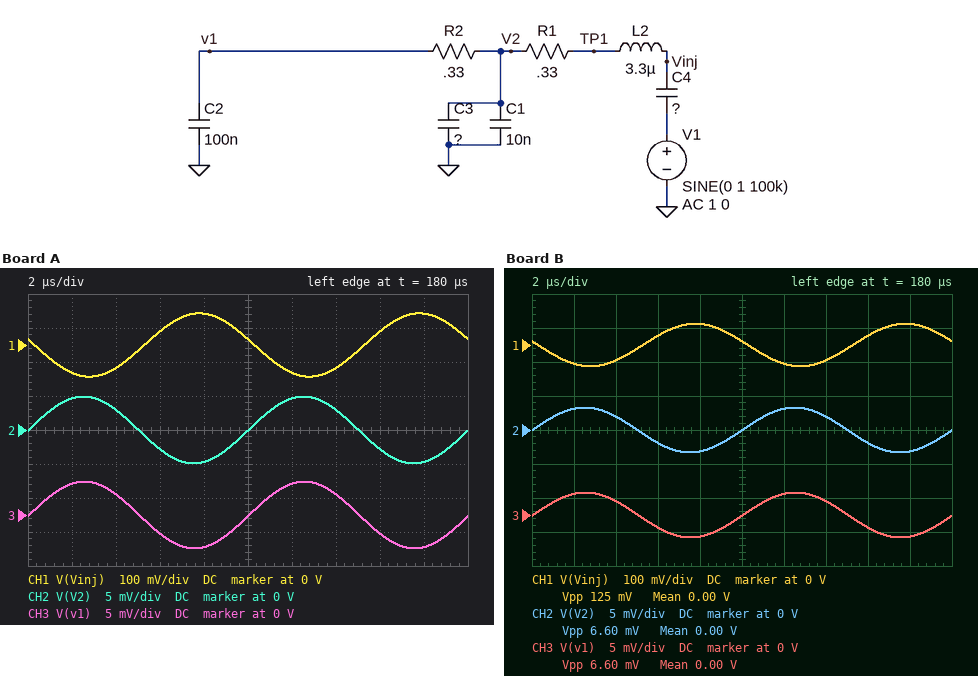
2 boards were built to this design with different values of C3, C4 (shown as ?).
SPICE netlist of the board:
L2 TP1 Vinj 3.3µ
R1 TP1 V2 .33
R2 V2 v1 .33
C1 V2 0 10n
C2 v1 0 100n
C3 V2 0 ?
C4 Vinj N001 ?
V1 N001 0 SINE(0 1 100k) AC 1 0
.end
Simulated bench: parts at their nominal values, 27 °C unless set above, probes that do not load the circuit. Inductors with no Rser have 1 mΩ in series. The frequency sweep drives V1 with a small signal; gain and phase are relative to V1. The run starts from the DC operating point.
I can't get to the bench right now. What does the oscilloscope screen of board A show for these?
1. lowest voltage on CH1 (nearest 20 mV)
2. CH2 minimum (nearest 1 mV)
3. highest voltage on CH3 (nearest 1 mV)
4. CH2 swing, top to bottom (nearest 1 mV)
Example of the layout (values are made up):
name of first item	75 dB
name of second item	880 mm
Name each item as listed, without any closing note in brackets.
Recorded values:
lowest voltage on CH1	-100 mV
CH2 minimum	-5 mV
highest voltage on CH3	5 mV
CH2 swing, top to bottom	10 mV
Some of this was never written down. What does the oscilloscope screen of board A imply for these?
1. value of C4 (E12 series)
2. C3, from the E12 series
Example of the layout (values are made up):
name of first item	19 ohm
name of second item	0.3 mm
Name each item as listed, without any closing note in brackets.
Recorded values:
value of C4	68 nF
C3, from the E12 series	15 µF
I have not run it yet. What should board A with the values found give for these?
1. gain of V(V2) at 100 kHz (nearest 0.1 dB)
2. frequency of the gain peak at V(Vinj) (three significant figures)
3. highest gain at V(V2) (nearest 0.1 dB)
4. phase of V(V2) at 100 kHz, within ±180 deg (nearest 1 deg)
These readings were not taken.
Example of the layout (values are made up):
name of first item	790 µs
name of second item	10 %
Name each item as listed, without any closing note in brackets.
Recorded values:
gain of V(V2) at 100 kHz	-46.2 dB
frequency of the gain peak at V(Vinj)	337 kHz
highest gain at V(V2)	-20.5 dB
phase of V(V2) at 100 kHz, within ±180 deg	-1 deg
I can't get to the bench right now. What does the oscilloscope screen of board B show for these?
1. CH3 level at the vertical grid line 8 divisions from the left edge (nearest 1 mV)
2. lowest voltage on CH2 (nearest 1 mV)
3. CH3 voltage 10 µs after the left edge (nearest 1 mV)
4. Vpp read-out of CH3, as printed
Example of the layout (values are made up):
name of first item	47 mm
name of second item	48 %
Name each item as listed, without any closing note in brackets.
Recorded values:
CH3 level at the vertical grid line 8 divisions from the left edge	-2 mV
lowest voltage on CH2	-3 mV
CH3 voltage 10 µs after the left edge	0 V
Vpp read-out of CH3, as printed	6.60 mV
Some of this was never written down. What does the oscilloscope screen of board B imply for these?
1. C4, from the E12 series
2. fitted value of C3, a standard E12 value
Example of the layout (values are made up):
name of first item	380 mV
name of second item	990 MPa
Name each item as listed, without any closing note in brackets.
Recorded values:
C4, from the E12 series	47 nF
fitted value of C3, a standard E12 value	15 µF
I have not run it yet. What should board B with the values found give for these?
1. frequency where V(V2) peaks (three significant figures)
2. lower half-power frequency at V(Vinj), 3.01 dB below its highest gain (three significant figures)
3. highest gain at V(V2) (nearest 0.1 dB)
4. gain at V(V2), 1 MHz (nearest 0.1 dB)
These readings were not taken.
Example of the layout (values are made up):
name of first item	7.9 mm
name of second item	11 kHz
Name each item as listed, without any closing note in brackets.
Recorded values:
frequency where V(V2) peaks	405 kHz
lower half-power frequency at V(Vinj), 3.01 dB below its highest gain	397 kHz
highest gain at V(V2)	-22.1 dB
gain at V(V2), 1 MHz	-64.3 dB
